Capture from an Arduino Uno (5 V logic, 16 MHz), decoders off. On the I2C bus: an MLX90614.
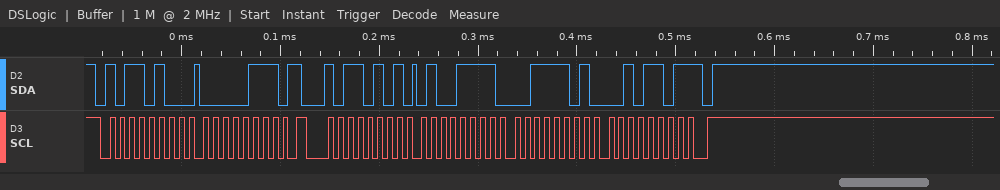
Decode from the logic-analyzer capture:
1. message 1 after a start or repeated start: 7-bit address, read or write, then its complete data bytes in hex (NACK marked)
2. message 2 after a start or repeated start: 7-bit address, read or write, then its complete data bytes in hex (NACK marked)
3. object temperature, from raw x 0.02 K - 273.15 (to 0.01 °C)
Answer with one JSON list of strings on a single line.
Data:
["0x5A write: 07", "0x5A read: 4F 3D 2D NACK", "40.75 °C"]
